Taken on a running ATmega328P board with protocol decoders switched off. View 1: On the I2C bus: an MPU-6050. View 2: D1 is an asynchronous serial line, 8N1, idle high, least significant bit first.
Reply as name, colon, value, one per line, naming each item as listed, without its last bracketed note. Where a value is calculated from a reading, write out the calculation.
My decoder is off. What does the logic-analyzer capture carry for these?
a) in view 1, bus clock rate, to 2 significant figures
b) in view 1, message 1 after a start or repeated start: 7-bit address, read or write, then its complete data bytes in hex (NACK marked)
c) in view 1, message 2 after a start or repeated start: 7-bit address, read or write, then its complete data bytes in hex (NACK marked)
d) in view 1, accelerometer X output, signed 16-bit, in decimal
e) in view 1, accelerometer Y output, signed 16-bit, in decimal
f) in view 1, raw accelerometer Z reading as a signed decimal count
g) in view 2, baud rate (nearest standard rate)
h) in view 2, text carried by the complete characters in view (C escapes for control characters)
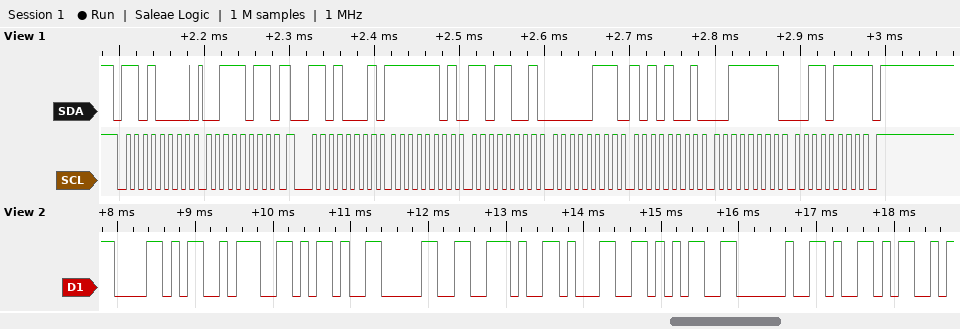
in view 1, bus clock rate, to 2 significant figures: 100 kHz
in view 1, message 1 after a start or repeated start: 7-bit address, read or write, then its complete data bytes in hex: 0x68 write: 3B
in view 1, message 2 after a start or repeated start: 7-bit address, read or write, then its complete data bytes in hex: 0x68 read: FD D9 07 A9 3F 37 NACK
in view 1, accelerometer X output, signed 16-bit, in decimal: 0xFDD9 = -551
in view 1, accelerometer Y output, signed 16-bit, in decimal: 0x07A9 = 1961
in view 1, raw accelerometer Z reading as a signed decimal count: 0x3F37 = 16183
in view 2, baud rate: 9600 baud
in view 2, text carried by the complete characters in view: "X:-0.15 Y"
